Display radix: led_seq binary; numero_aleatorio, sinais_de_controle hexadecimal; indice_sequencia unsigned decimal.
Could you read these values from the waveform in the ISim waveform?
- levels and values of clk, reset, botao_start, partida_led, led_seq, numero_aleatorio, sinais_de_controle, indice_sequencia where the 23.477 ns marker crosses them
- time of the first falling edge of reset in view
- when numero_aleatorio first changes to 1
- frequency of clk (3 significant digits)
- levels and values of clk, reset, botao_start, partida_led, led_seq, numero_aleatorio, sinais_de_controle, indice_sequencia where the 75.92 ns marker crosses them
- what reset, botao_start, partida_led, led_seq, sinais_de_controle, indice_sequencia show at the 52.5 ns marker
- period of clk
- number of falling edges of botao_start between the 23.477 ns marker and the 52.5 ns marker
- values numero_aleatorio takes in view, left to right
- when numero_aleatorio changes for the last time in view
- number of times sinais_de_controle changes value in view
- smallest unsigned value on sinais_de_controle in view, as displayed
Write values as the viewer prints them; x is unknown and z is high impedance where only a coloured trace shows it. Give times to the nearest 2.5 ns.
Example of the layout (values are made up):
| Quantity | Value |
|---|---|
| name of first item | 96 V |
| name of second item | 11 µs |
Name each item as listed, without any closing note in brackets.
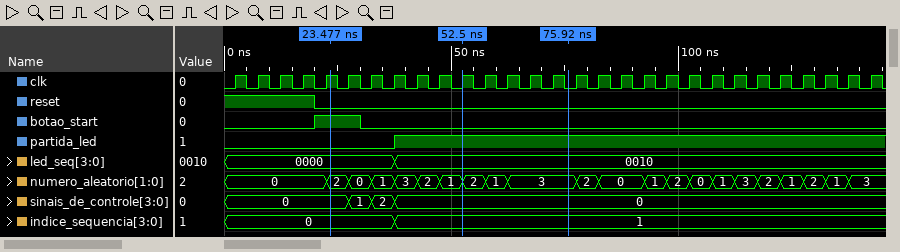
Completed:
| Quantity | Value |
|---|---|
| levels and values of clk, reset, botao_start, partida_led, led_seq, numero_aleatorio, sinais_de_controle, indice_sequencia where the 23.477 ns marker crosses them | clk=1, reset=0, botao_start=1, partida_led=0, led_seq=0000, numero_aleatorio=2, sinais_de_controle=0, indice_sequencia=0 |
| time of the first falling edge of reset in view | 20 ns |
| when numero_aleatorio first changes to 1 | 32.5 ns |
| frequency of clk | 200 MHz |
| levels and values of clk, reset, botao_start, partida_led, led_seq, numero_aleatorio, sinais_de_controle, indice_sequencia where the 75.92 ns marker crosses them | clk=0, reset=0, botao_start=0, partida_led=1, led_seq=0010, numero_aleatorio=3, sinais_de_controle=0, indice_sequencia=1 |
| what reset, botao_start, partida_led, led_seq, sinais_de_controle, indice_sequencia show at the 52.5 ns marker | reset=0, botao_start=0, partida_led=1, led_seq=0010, sinais_de_controle=0, indice_sequencia=1 |
| period of clk | 5 ns |
| number of falling edges of botao_start between the 23.477 ns marker and the 52.5 ns marker | 1 |
| values numero_aleatorio takes in view, left to right | 0, 2, 0, 1, 3, 2, 1, 2, 1, 3, 2, 0, 1, 2, 0, 1, 3, 2, 1, 2, 1, 3 |
| when numero_aleatorio changes for the last time in view | 137.5 ns |
| number of times sinais_de_controle changes value in view | 3 |
| smallest unsigned value on sinais_de_controle in view, as displayed | 0 |
